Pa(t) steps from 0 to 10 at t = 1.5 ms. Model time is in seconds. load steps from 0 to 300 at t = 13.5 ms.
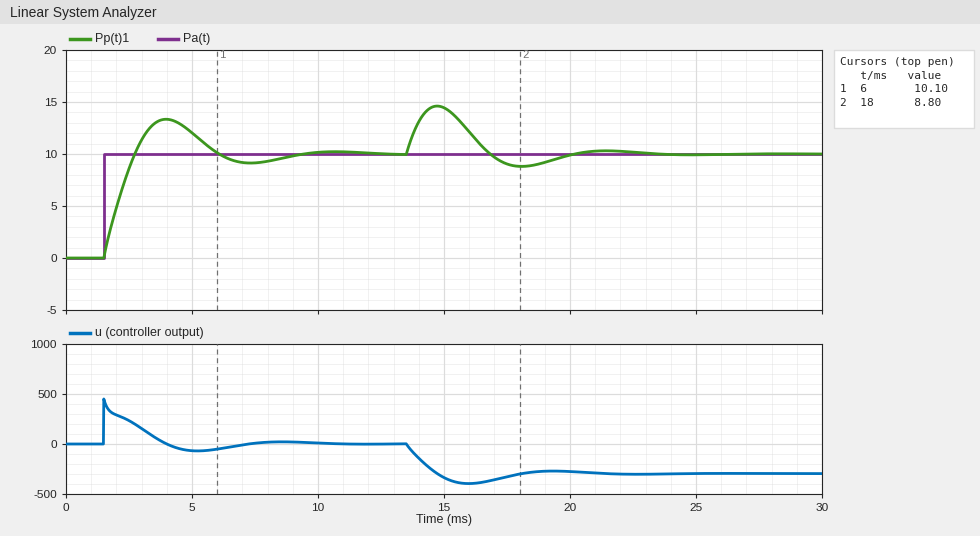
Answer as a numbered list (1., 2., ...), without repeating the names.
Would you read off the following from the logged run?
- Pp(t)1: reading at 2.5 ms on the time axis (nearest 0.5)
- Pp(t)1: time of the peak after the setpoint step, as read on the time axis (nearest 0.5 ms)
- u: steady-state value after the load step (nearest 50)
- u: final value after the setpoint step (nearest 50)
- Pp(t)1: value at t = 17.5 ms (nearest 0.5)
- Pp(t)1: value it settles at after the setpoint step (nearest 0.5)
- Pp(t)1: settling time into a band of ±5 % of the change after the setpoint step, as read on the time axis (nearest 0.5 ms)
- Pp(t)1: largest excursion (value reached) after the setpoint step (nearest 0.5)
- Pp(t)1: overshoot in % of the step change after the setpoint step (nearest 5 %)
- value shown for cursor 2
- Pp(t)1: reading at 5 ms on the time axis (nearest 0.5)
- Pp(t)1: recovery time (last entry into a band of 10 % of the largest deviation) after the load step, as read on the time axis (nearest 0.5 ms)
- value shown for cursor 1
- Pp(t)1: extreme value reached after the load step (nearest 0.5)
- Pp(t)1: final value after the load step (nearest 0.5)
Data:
1. 8.5
2. 4.0 ms
3. -300
4. 0
5. 9.0
6. 10.0
7. 8.5 ms
8. 13.5
9. 35 %
10. 8.80
11. 12.0
12. 19.5 ms
13. 10.10
14. 14.5
15. 10.0
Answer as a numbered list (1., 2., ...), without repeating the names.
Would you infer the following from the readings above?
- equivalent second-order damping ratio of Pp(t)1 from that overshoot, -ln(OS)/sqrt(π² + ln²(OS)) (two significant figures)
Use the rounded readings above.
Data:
1. 0.32
